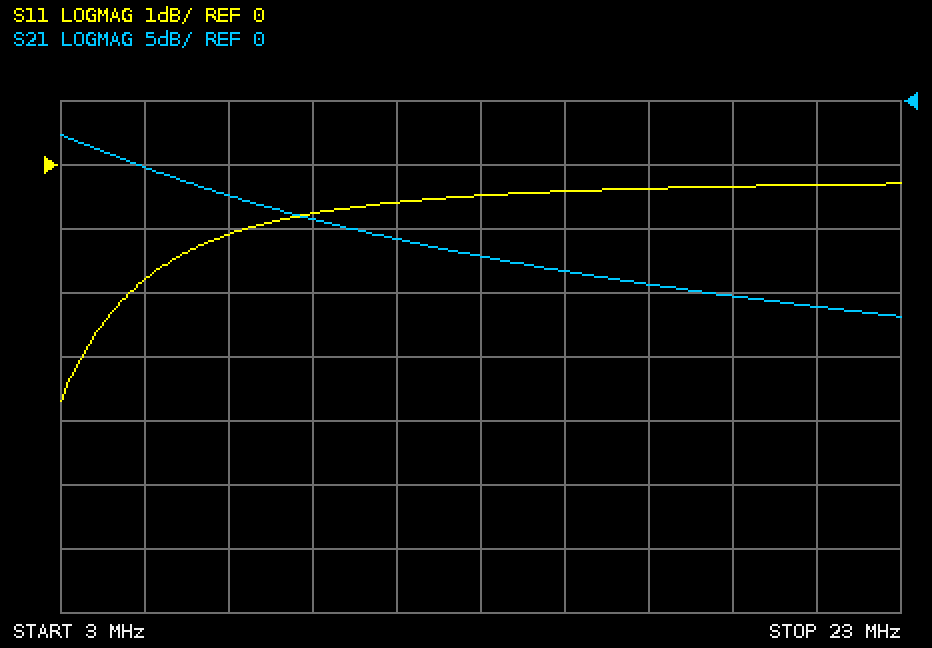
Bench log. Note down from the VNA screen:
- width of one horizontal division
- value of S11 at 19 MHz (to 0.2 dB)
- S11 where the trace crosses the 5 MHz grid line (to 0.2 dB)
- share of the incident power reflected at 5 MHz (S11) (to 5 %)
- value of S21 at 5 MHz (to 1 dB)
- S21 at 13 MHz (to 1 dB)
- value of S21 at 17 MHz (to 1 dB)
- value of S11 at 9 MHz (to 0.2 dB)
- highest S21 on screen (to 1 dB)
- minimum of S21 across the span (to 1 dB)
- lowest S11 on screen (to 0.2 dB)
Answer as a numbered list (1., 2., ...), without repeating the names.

1. 2 MHz
2. -0.4 dB
3. -1.8 dB
4. 65 %
5. -5 dB
6. -12 dB
7. -14 dB
8. -0.8 dB
9. -3 dB
10. -17 dB
11. -3.6 dB
